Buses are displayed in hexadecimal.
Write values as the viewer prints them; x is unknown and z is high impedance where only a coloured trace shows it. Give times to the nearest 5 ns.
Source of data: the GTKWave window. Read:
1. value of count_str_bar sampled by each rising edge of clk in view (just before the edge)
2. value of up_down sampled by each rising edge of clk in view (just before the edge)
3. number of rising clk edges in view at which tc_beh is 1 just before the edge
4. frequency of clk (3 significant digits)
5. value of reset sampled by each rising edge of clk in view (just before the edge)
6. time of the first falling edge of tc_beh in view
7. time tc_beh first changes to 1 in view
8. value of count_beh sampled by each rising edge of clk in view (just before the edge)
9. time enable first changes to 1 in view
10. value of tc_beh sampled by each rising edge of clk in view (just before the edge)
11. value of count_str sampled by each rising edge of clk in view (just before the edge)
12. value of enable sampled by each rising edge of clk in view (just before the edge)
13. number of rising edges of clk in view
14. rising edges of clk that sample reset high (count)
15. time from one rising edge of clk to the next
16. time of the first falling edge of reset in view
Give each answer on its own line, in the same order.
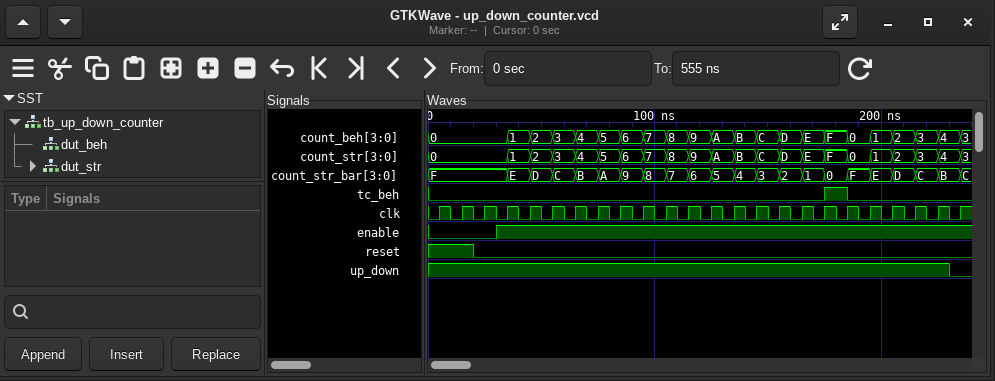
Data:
F, F, F, F, E, D, C, B, A, 9, 8, 7, 6, 5, 4, 3, 2, 1, 0, F, E, D, C, B
1 1 1 1 1 1 1 1 1 1 1 1 1 1 1 1 1 1 1 1 1 1 1 0
1
100 MHz
1 1 0 0 0 0 0 0 0 0 0 0 0 0 0 0 0 0 0 0 0 0 0 0
185 ns
175 ns
0, 0, 0, 0, 1, 2, 3, 4, 5, 6, 7, 8, 9, A, B, C, D, E, F, 0, 1, 2, 3, 4
30 ns
0 0 0 0 0 0 0 0 0 0 0 0 0 0 0 0 0 0 1 0 0 0 0 0
0, 0, 0, 0, 1, 2, 3, 4, 5, 6, 7, 8, 9, A, B, C, D, E, F, 0, 1, 2, 3, 4
0 0 0 1 1 1 1 1 1 1 1 1 1 1 1 1 1 1 1 1 1 1 1 1
24
2
10 ns
20 ns
